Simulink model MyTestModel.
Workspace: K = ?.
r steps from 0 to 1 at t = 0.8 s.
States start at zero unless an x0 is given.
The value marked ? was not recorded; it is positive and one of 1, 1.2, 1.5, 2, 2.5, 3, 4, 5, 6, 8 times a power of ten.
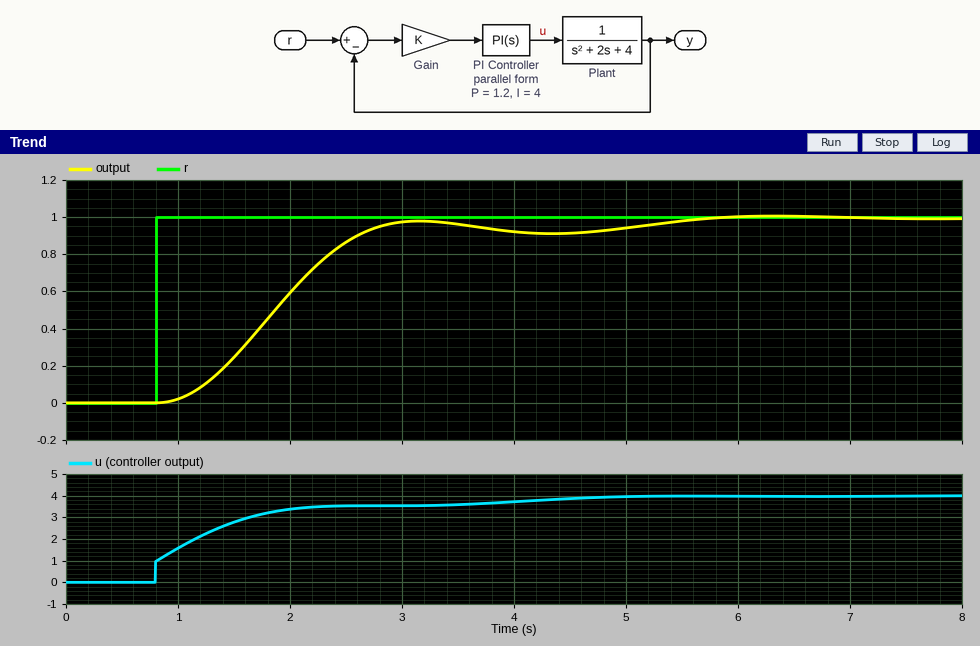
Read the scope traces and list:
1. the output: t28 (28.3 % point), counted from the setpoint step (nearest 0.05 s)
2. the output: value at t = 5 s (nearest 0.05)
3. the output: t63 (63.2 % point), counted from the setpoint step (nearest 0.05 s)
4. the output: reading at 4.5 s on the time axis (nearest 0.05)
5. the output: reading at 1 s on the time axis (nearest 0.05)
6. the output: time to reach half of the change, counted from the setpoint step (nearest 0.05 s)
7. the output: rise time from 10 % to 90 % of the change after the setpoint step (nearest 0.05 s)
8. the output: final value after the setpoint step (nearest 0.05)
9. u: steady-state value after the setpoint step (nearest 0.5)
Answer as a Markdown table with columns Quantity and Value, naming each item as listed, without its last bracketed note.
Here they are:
| Quantity | Value |
|---|---|
| the output: t28 (28.3 % point), counted from the setpoint step | 0.75 s |
| the output: value at t = 5 s | 0.95 |
| the output: t63 (63.2 % point), counted from the setpoint step | 1.25 s |
| the output: reading at 4.5 s on the time axis | 0.90 |
| the output: reading at 1 s on the time axis | 0.00 |
| the output: time to reach half of the change, counted from the setpoint step | 1.05 s |
| the output: rise time from 10 % to 90 % of the change after the setpoint step | 1.35 s |
| the output: final value after the setpoint step | 1.00 |
| u: steady-state value after the setpoint step | 4.0 |
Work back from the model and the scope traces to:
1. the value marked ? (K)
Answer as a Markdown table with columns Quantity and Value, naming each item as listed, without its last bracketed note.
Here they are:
| Quantity | Value |
|---|---|
| the value marked ? | 0.8 |
